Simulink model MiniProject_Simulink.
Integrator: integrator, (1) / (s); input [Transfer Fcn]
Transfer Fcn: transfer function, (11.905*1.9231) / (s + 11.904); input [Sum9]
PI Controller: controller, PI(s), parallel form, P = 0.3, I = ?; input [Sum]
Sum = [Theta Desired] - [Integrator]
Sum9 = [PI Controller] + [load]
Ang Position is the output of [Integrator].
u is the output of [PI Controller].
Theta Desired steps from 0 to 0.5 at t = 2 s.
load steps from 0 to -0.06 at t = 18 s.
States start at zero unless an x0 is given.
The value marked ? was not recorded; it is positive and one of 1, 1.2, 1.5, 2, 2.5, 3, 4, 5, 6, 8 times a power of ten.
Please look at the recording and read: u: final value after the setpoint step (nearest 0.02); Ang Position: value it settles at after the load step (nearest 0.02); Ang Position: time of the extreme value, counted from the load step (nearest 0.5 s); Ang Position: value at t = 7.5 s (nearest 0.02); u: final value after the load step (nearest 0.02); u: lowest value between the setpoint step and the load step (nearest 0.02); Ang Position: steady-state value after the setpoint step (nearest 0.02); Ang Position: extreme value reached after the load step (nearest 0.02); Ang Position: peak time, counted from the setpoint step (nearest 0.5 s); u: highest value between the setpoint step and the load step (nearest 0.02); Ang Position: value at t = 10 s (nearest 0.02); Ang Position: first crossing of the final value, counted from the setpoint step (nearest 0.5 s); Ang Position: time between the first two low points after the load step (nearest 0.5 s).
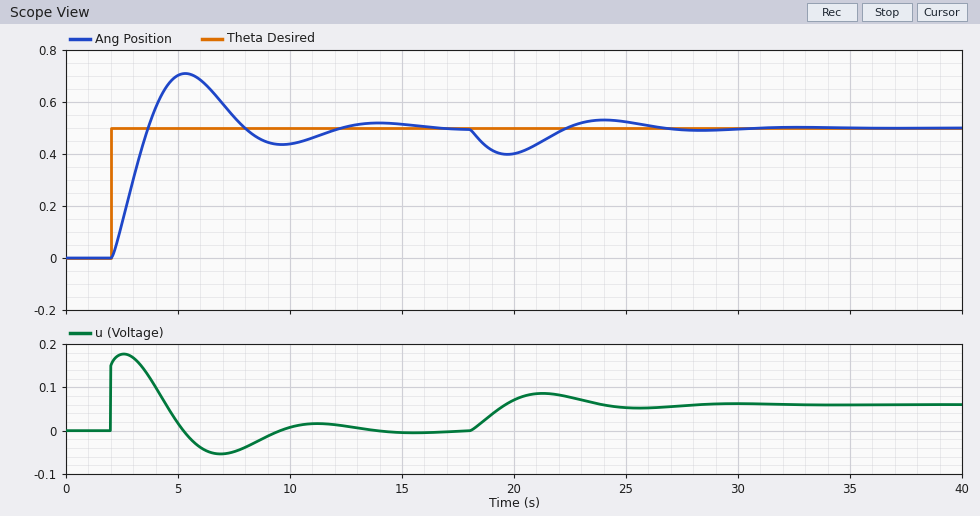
0.00
0.50
1.5 s
0.54
0.06
-0.06
0.50
0.40
3.5 s
0.18
0.44
1.5 s
8.5 s
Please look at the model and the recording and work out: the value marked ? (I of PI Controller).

0.3
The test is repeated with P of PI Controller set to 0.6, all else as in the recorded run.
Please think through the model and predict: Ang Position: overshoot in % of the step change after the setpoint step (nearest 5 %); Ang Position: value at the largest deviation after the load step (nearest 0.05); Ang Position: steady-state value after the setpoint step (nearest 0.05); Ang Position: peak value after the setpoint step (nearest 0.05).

20 %
0.45
0.50
0.60
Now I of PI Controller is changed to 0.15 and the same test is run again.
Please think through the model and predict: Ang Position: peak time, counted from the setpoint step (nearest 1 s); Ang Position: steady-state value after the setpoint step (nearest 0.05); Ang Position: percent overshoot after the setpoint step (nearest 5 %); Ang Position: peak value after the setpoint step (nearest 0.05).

4 s
0.50
30 %
0.65
